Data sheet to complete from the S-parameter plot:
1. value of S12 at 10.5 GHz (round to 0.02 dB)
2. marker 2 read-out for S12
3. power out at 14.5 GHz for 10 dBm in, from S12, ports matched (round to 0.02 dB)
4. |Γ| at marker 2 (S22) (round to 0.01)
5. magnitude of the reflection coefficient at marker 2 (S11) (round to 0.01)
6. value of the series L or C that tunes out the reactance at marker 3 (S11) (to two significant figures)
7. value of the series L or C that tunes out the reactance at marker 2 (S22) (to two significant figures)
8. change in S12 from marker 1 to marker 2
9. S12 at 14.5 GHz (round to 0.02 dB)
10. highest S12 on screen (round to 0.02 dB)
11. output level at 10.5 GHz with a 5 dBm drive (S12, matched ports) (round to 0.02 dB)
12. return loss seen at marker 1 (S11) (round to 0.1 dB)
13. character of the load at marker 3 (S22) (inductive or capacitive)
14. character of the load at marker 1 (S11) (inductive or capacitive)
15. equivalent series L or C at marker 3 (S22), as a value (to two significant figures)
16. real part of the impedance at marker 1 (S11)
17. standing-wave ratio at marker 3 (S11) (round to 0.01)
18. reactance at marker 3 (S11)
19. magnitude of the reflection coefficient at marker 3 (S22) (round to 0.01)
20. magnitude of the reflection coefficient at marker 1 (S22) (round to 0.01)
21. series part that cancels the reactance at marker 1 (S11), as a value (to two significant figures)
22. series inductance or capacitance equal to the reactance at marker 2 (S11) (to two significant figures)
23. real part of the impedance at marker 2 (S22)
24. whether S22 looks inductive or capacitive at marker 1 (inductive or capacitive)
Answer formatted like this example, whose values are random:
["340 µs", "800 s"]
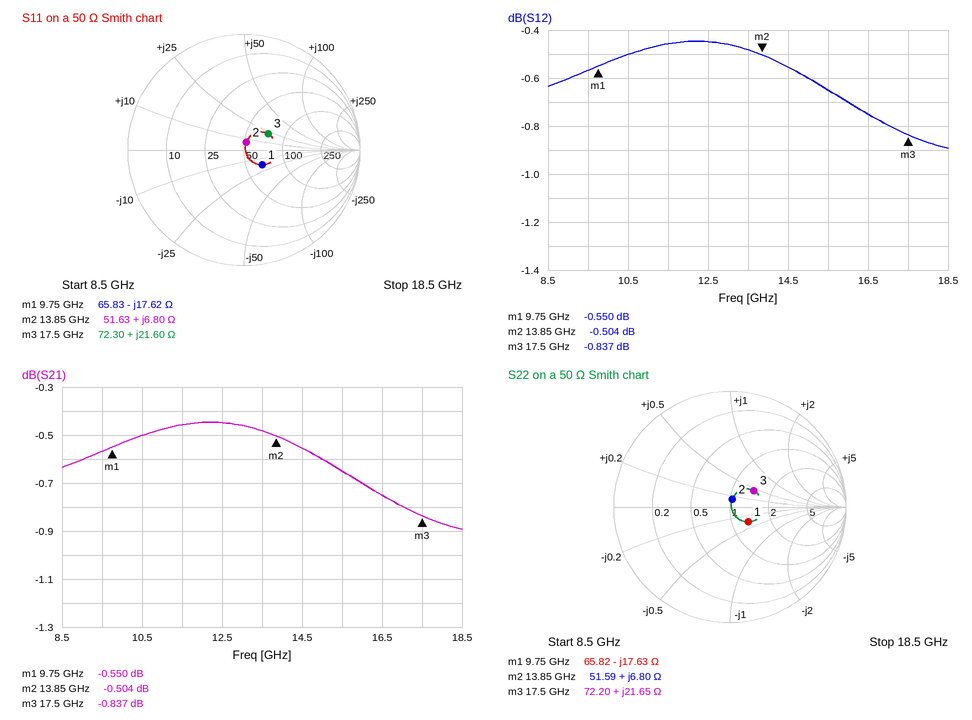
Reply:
["-0.50 dB", "-0.504 dB", "9.44 dBm", "0.07", "0.07", "420 fF", "1.7 pF", "0.046 dB", "-0.56 dB", "-0.44 dB", "4.50 dBm", "13.9 dB", "inductive", "capacitive", "200 pH", "65.83 Ω", "1.67", "+21.60 Ω", "0.25", "0.20", "290 pH", "78 pH", "51.59 Ω", "capacitive"]
